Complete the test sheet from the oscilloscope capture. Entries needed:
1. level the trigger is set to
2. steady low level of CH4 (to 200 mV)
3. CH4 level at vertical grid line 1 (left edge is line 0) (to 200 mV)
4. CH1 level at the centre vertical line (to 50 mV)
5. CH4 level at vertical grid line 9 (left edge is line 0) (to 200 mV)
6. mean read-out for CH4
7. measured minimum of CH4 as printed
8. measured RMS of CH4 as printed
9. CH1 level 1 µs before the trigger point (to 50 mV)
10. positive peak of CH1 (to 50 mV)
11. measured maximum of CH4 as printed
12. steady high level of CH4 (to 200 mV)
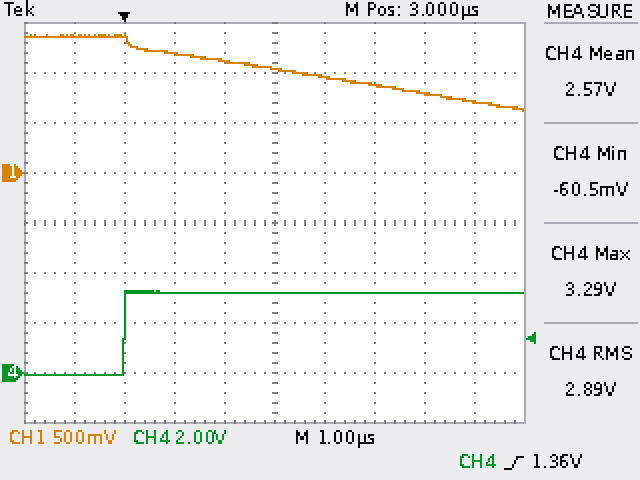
1.36 V
0.0 V
0.0 V
1.05 V
3.2 V
2.57 V
-60.5 mV
2.89 V
1.35 V
1.40 V
3.29 V
3.2 V
